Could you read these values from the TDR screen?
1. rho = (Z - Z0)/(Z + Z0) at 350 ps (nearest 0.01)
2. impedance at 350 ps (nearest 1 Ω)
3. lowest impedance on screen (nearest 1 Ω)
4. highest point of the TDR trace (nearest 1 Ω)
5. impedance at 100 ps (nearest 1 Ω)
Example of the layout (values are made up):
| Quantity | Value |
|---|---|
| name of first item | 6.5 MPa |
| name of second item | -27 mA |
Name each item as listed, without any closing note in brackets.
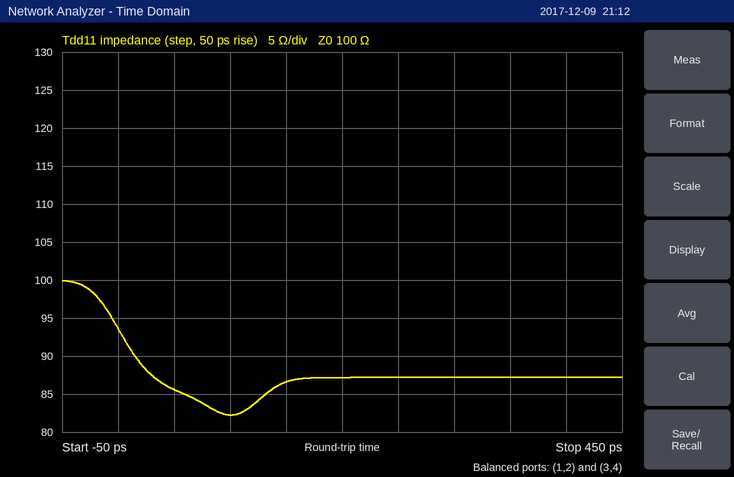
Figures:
| Quantity | Value |
|---|---|
| rho = (Z - Z0)/(Z + Z0) at 350 ps | -0.07 |
| impedance at 350 ps | 87 Ω |
| lowest impedance on screen | 82 Ω |
| highest point of the TDR trace | 100 Ω |
| impedance at 100 ps | 82 Ω |
